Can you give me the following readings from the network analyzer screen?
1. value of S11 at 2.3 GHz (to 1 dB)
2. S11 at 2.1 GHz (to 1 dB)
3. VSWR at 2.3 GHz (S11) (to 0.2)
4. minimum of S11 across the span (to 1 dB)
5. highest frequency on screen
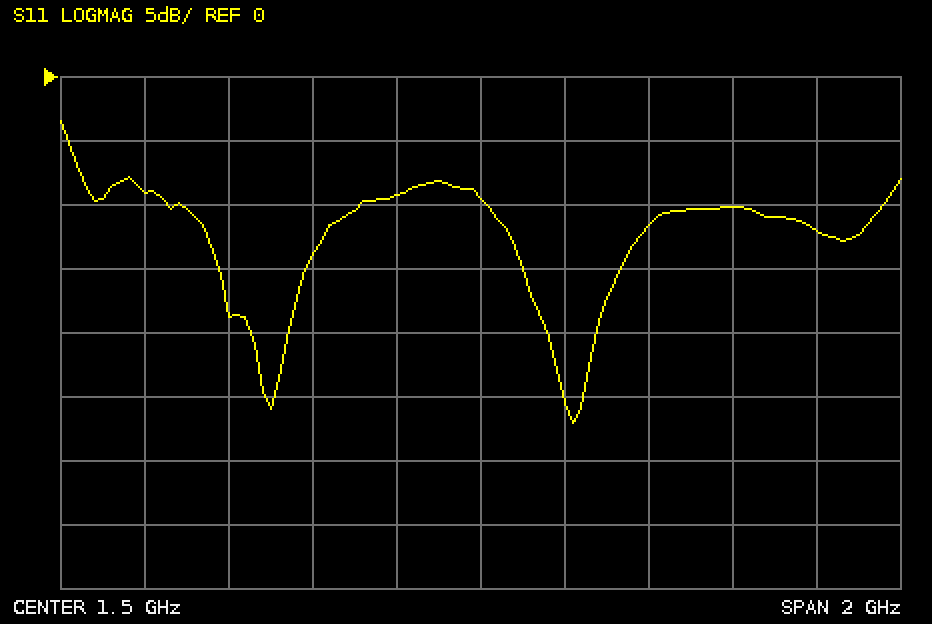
-12 dB
-10 dB
1.6
-27 dB
2.5 GHz
